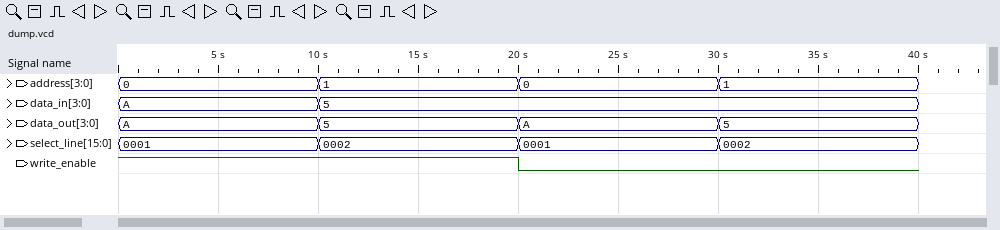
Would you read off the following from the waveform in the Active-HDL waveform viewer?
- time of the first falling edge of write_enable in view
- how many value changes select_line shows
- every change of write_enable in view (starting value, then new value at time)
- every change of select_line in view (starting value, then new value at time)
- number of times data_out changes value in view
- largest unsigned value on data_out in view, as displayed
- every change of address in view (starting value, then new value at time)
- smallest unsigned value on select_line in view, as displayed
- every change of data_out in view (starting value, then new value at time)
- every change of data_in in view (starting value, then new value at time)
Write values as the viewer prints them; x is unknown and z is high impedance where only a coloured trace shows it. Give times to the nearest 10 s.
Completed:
20 s
3
1, 0 at 20 s
0001, 0002 at 10 s, 0001 at 20 s, 0002 at 30 s
3
A
0, 1 at 10 s, 0 at 20 s, 1 at 30 s
0001
A, 5 at 10 s, A at 20 s, 5 at 30 s
A, 5 at 10 s
